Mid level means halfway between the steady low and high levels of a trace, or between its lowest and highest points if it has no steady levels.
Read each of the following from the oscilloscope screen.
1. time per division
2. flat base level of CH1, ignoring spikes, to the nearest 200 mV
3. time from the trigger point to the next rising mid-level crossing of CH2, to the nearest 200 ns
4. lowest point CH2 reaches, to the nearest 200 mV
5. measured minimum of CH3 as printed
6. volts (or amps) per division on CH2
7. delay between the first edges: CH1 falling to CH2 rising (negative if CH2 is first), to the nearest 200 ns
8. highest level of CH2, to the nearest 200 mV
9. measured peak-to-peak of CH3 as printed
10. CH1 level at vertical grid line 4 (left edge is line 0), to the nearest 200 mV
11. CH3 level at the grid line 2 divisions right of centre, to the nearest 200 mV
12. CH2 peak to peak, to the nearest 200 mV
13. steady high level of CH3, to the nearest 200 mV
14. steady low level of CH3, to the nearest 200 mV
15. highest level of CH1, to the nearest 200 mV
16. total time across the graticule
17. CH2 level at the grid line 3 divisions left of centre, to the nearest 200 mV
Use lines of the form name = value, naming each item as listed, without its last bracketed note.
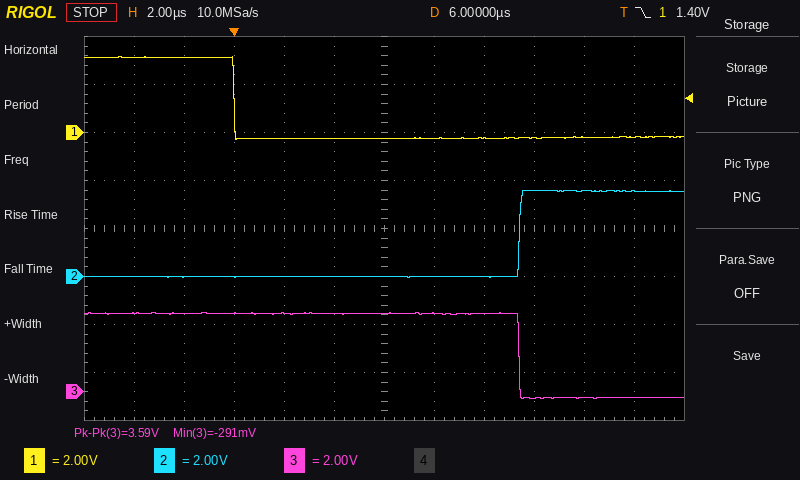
time per division = 2 µs
flat base level of CH1, ignoring spikes, to the nearest 200 mV = -200 mV
time from the trigger point to the next rising mid-level crossing of CH2, to the nearest 200 ns = 11.4 µs
lowest point CH2 reaches, to the nearest 200 mV = 0.0 V
measured minimum of CH3 as printed = -291 mV
volts (or amps) per division on CH2 = 2 V
delay between the first edges: CH1 falling to CH2 rising (negative if CH2 is first), to the nearest 200 ns = +11.4 µs
highest level of CH2, to the nearest 200 mV = 3.6 V
measured peak-to-peak of CH3 as printed = 3.59 V
CH1 level at vertical grid line 4 (left edge is line 0), to the nearest 200 mV = -200 mV
CH3 level at the grid line 2 divisions right of centre, to the nearest 200 mV = 3.2 V
CH2 peak to peak, to the nearest 200 mV = 3.6 V
steady high level of CH3, to the nearest 200 mV = 3.2 V
steady low level of CH3, to the nearest 200 mV = -200 mV
highest level of CH1, to the nearest 200 mV = 3.2 V
total time across the graticule = 24 µs
CH2 level at the grid line 3 divisions left of centre, to the nearest 200 mV = 0.0 V
